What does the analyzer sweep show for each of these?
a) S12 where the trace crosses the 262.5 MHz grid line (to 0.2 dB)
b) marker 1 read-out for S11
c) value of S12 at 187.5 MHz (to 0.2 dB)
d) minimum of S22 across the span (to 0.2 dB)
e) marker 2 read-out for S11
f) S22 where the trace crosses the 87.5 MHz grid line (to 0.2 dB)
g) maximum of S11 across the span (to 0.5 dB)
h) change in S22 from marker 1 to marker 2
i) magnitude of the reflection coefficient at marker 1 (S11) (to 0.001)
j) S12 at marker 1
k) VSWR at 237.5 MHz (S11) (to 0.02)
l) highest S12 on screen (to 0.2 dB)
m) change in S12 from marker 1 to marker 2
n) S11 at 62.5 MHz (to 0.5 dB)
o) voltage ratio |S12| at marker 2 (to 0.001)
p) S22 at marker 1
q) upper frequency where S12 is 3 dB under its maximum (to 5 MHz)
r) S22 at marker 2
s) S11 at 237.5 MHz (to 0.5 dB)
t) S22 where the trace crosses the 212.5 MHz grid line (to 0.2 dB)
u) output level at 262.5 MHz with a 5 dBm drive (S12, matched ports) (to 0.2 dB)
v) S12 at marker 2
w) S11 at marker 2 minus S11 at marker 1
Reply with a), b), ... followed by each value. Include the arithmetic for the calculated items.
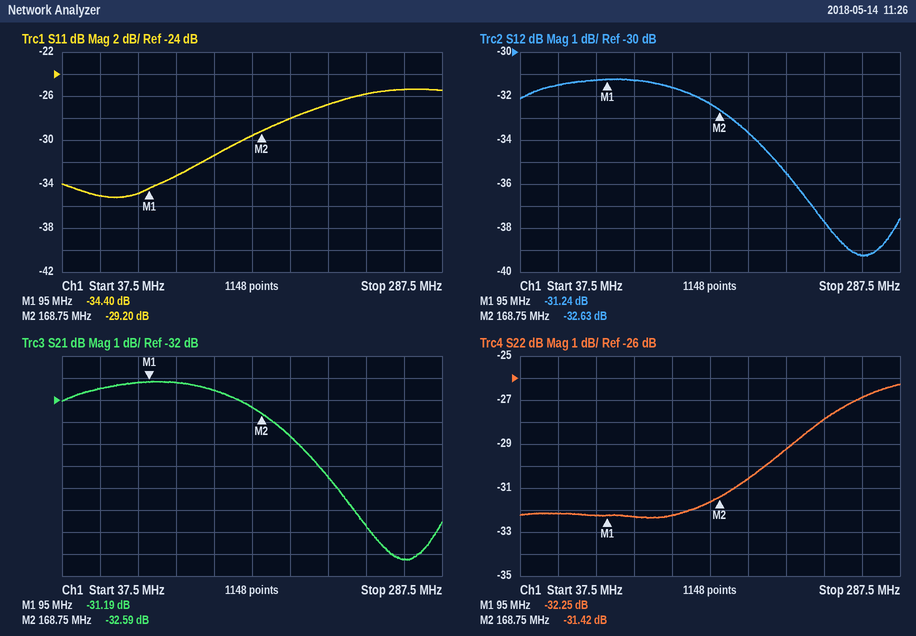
a) -39.2 dB
b) -34.40 dB
c) -33.6 dB
d) -32.4 dB
e) -29.20 dB
f) -32.2 dB
g) -25.5 dB
h) -31.42 − (-32.25) = 0.83 dB
i) 10^(-34.4/20) ≈ 0.019
j) -31.24 dB
k) |Γ| = 10^(-26/20) = 0.0501; VSWR = (1 + 0.0501)/(1 − 0.0501) ≈ 1.11, so 1.10 to the nearest 0.02
l) -31.2 dB
m) -32.63 − (-31.24) = -1.39 dB
n) -35.0 dB
o) 10^(-32.63/20) ≈ 0.023
p) -32.25 dB
q) 195 MHz
r) -31.42 dB
s) -26.0 dB
t) -29.2 dB
u) 5 dBm + (-39.2 dB) = -34.2 dBm
v) -32.63 dB
w) -29.2 − (-34.4) = 5.20 dB
